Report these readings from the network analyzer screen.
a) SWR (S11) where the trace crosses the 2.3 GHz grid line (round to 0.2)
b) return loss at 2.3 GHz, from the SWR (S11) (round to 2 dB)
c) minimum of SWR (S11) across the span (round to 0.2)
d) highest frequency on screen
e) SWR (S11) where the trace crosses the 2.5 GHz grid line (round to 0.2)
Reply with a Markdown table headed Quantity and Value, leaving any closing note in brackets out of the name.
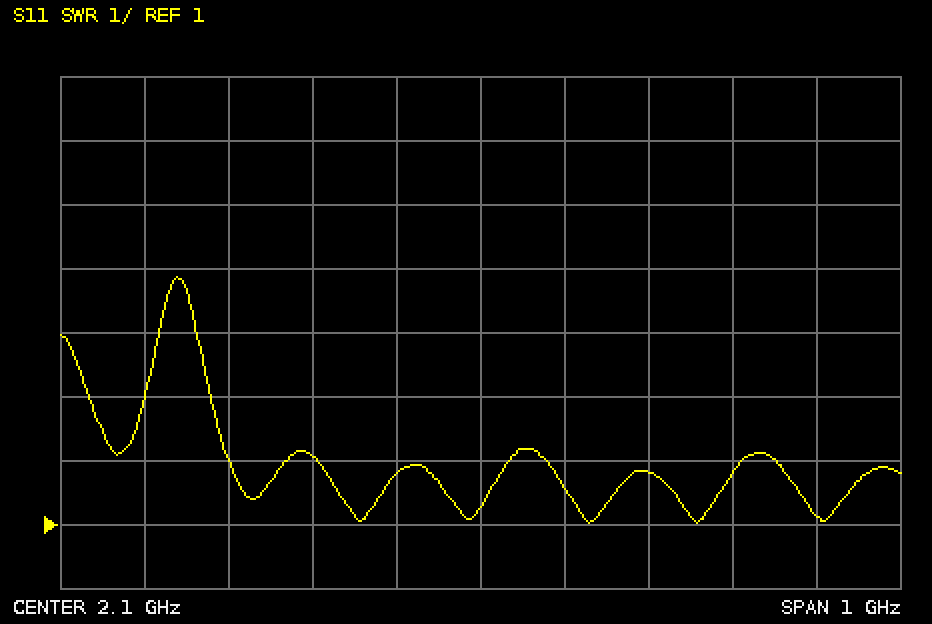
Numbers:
| Quantity | Value |
|---|---|
| SWR (S11) where the trace crosses the 2.3 GHz grid line | 1.8 |
| return loss at 2.3 GHz, from the SWR (S11) | 10 dB |
| minimum of SWR (S11) across the span | 1.0 |
| highest frequency on screen | 2.6 GHz |
| SWR (S11) where the trace crosses the 2.5 GHz grid line | 1.2 |
